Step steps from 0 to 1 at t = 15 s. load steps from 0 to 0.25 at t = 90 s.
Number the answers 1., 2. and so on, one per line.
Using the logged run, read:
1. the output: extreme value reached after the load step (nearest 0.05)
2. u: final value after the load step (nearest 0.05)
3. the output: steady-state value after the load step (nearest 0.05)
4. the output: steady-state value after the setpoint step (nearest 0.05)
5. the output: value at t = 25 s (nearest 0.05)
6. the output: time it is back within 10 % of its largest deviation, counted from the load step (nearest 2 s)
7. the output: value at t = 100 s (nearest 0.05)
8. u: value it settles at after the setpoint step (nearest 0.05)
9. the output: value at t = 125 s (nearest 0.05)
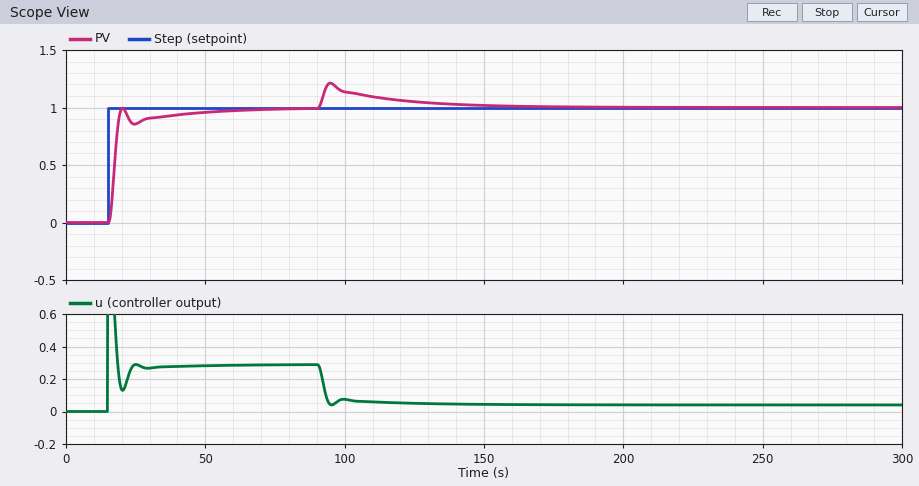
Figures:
1. 1.20
2. 0.05
3. 1.00
4. 1.00
5. 0.85
6. 54 s
7. 1.15
8. 0.30
9. 1.05
